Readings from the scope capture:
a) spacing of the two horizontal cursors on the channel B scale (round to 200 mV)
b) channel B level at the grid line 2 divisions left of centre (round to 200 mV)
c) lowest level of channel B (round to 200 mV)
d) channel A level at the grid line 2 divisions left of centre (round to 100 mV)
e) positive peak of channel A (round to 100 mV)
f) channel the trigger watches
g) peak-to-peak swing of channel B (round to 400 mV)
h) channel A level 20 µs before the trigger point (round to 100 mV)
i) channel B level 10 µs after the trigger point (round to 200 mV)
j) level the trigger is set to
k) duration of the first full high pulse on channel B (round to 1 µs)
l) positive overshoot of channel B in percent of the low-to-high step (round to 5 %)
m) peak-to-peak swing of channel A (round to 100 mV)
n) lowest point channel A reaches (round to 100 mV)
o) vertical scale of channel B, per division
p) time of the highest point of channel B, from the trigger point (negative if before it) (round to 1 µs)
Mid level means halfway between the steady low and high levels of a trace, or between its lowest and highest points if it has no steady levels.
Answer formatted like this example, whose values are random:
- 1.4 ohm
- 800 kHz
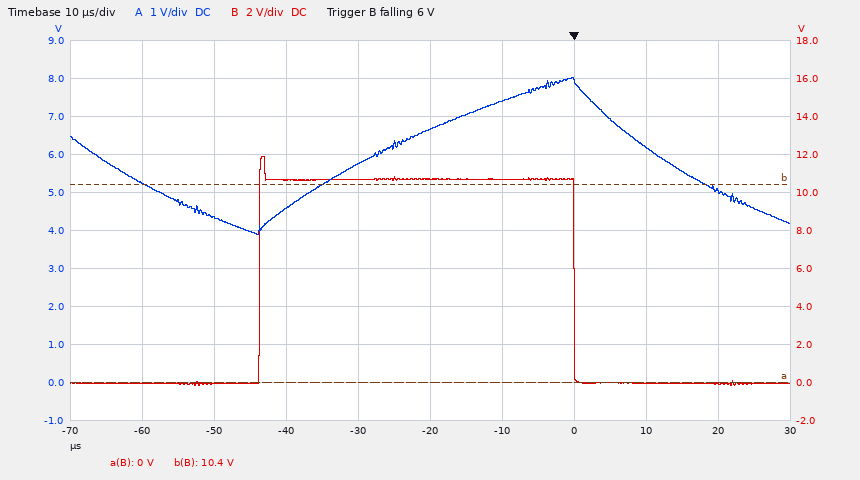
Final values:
- 10.4 V
- 10.6 V
- -200 mV
- 4.6 V
- 8.0 V
- channel B
- 12.0 V
- 6.7 V
- 0.0 V
- 6 V
- 44 µs
- 10 %
- 4.1 V
- 3.9 V
- 2 V
- -43 µs
